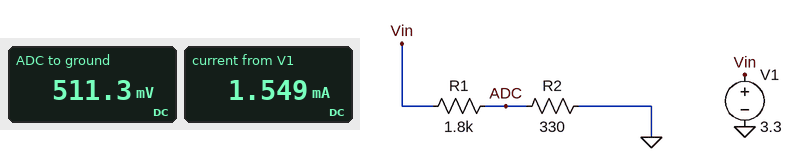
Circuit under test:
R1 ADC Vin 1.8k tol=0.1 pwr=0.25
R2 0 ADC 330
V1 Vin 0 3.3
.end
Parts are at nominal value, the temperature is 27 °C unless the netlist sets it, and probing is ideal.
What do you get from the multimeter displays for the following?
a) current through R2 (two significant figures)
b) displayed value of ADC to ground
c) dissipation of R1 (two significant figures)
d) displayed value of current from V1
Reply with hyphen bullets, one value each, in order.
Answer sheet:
- 1.5 mA
- 511.3 mV
- 4.3 mW
- 1.549 mA
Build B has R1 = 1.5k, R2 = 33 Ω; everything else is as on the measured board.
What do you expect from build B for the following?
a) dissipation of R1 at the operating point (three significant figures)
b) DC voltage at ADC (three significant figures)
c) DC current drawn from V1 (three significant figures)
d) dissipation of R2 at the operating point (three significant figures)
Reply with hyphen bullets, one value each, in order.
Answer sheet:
- 6.95 mW
- 71.0 mV
- 2.15 mA
- 153 µW
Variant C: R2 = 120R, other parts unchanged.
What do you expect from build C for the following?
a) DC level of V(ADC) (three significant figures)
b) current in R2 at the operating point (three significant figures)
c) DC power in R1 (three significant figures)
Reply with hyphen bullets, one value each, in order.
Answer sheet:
- 206 mV
- 1.72 mA
- 5.32 mW
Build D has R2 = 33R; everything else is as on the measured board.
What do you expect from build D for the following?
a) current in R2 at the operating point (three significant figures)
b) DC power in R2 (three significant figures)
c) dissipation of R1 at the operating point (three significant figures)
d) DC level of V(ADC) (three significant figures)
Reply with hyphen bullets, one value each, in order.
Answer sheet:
- 1.80 mA
- 107 µW
- 5.83 mW
- 59.4 mV
